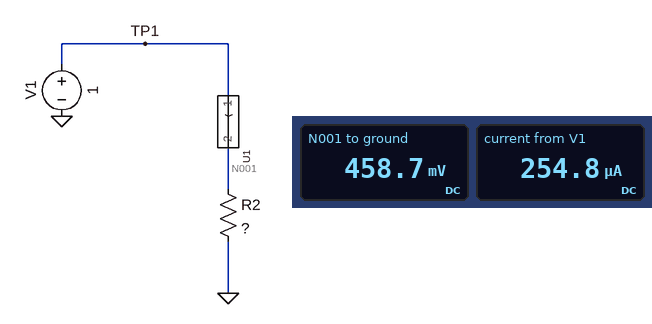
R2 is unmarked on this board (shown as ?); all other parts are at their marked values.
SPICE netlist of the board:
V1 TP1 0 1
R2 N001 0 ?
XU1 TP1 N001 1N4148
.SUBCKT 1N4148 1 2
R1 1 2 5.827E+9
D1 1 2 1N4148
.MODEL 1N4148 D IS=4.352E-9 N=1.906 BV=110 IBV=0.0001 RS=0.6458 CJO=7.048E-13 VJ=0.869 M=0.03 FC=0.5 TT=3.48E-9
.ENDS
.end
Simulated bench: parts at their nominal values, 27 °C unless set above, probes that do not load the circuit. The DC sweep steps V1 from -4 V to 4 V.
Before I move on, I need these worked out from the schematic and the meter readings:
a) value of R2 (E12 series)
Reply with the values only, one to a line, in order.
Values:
1.8 kΩ
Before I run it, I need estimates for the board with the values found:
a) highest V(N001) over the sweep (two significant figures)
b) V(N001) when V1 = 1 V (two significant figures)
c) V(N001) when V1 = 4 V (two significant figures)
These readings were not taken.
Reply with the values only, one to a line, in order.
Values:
3.4 V
460 mV
3.4 V
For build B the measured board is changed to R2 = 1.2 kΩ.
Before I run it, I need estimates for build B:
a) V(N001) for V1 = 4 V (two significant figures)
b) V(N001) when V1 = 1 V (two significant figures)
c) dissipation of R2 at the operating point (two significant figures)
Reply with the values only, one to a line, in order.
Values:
3.3 V
440 mV
160 µW
